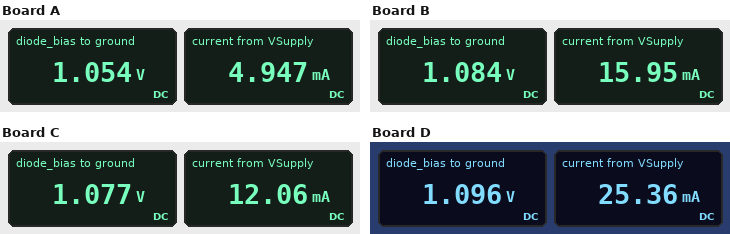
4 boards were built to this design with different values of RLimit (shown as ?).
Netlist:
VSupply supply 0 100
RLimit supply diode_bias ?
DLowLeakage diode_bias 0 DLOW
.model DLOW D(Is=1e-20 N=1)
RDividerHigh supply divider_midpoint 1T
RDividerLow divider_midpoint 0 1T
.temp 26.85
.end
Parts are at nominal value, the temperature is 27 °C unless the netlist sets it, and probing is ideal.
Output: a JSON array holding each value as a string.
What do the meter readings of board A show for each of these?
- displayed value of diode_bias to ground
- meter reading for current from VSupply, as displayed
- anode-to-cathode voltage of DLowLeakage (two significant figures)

["1.054 V", "4.947 mA", "1.1 V"]
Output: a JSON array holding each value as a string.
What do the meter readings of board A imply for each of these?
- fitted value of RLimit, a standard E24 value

["20 kΩ"]
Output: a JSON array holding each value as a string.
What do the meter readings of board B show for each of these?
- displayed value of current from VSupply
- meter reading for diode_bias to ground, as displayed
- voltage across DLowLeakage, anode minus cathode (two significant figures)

["15.95 mA", "1.084 V", "1.1 V"]
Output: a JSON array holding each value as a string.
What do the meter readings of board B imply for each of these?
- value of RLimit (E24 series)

["6.2 kΩ"]
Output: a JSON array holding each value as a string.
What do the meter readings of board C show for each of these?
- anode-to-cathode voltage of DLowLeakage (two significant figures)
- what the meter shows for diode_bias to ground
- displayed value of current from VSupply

["1.1 V", "1.077 V", "12.06 mA"]
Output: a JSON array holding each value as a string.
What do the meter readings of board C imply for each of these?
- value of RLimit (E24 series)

["8.2 kΩ"]
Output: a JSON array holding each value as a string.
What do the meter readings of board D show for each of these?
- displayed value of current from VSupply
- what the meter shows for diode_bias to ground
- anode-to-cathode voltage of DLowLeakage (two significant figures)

["25.36 mA", "1.096 V", "1.1 V"]
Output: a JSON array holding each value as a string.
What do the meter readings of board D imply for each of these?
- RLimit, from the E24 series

["3.9 kΩ"]
